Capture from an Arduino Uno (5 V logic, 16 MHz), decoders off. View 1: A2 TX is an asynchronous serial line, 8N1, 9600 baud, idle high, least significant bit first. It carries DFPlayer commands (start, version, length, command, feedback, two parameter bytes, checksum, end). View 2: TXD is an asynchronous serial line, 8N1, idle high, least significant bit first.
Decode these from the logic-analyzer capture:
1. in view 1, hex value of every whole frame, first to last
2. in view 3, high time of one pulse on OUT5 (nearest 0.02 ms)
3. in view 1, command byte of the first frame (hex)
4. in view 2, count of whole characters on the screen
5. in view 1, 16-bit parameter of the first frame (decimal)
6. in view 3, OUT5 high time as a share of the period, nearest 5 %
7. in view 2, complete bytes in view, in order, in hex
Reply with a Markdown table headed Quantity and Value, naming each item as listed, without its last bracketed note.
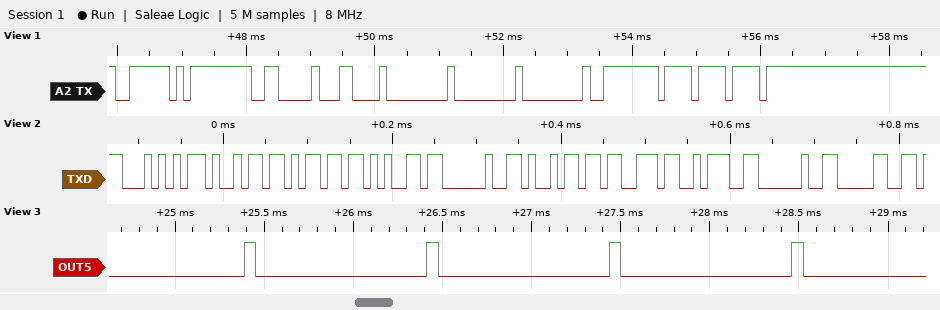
| Quantity | Value |
|---|---|
| in view 1, hex value of every whole frame, first to last | 7E FF 06 0C 00 00 00 FE EF EF |
| in view 3, high time of one pulse on OUT5 | 0.06 ms |
| in view 1, command byte of the first frame | 0x0C |
| in view 2, count of whole characters on the screen | 10 |
| in view 1, 16-bit parameter of the first frame | 0 |
| in view 3, OUT5 high time as a share of the period, nearest 5 % | 5 % |
| in view 2, complete bytes in view, in order, in hex | 54 69 6D 65 20 69 73 3A 20 30 |
